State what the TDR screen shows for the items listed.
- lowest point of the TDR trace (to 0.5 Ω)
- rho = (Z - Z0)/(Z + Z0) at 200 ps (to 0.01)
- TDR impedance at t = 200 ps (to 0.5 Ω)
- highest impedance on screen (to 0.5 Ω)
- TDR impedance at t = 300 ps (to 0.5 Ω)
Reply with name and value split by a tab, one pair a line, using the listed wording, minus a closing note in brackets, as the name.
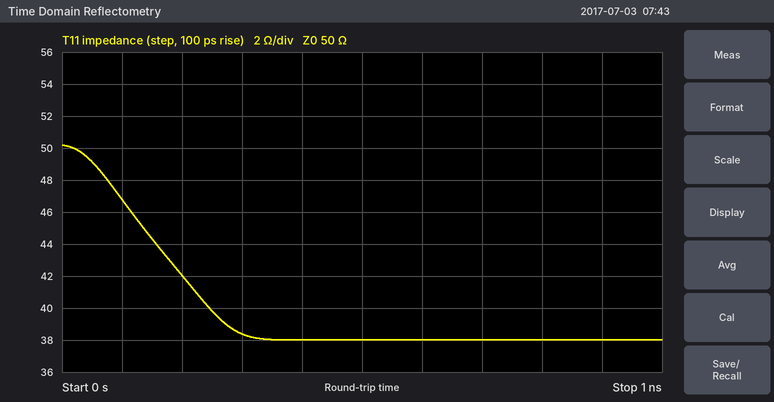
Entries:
lowest point of the TDR trace	38.0 Ω
rho = (Z - Z0)/(Z + Z0) at 200 ps	-0.09
TDR impedance at t = 200 ps	42.0 Ω
highest impedance on screen	50.0 Ω
TDR impedance at t = 300 ps	38.5 Ω
